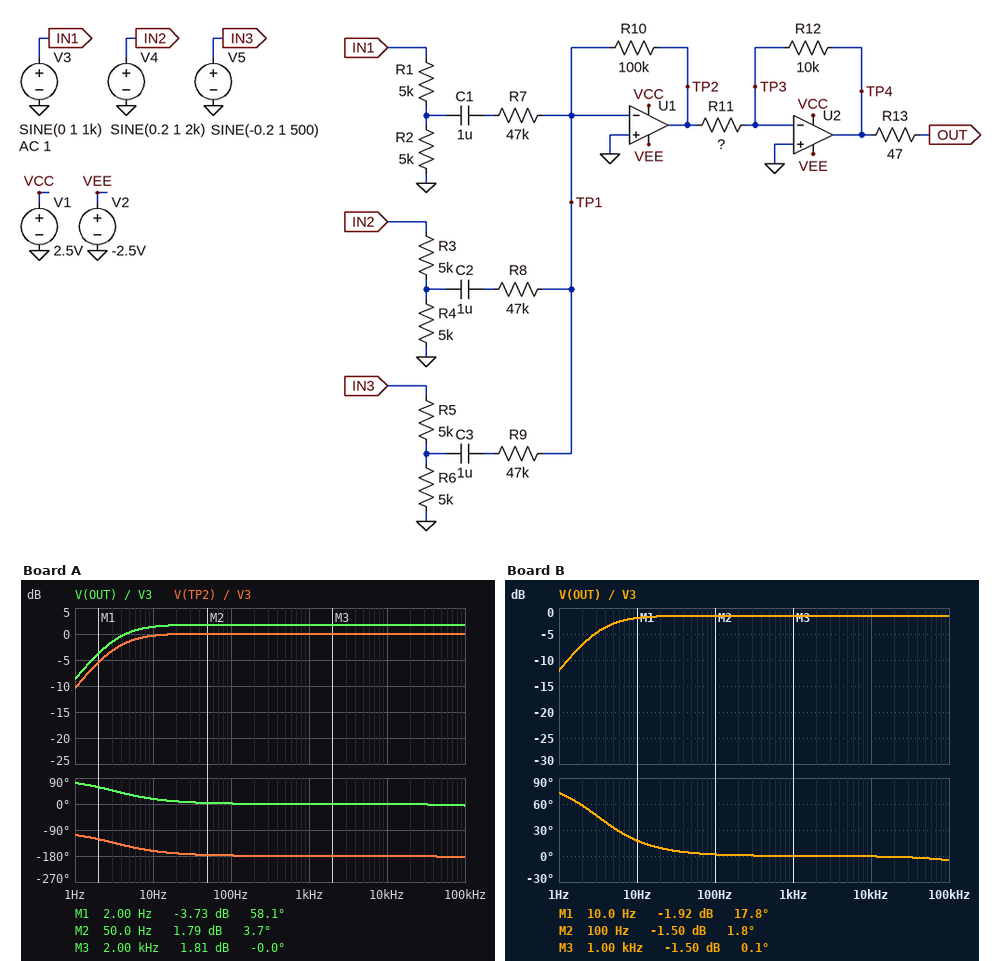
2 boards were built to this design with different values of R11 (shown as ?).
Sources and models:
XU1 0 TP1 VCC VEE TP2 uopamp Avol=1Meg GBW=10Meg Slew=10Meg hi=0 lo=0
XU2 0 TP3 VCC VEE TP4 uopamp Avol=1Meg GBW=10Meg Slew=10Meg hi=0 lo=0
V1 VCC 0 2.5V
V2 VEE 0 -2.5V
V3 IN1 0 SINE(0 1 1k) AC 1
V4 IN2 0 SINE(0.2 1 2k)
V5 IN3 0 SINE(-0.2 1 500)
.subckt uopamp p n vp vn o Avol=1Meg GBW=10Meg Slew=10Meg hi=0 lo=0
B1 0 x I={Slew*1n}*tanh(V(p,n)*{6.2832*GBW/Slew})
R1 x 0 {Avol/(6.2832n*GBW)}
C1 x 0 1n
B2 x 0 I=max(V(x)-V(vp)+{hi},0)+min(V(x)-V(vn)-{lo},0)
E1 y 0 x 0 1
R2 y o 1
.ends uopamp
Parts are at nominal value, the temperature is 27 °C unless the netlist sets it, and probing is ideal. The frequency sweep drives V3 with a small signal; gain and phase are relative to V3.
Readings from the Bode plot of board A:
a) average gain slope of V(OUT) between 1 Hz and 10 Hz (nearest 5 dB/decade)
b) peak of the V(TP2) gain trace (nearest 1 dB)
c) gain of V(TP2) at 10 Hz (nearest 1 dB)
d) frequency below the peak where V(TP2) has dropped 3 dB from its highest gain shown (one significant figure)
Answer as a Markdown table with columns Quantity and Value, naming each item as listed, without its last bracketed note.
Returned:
| Quantity | Value |
|---|---|
| average gain slope of V(OUT) between 1 Hz and 10 Hz | 10 dB/decade |
| peak of the V(TP2) gain trace | 0 dB |
| gain of V(TP2) at 10 Hz | 0 dB |
| frequency below the peak where V(TP2) has dropped 3 dB from its highest gain shown | 3 Hz |
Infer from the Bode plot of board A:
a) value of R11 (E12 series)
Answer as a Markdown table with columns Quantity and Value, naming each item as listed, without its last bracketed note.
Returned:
| Quantity | Value |
|---|---|
| value of R11 | 8.2 kΩ |
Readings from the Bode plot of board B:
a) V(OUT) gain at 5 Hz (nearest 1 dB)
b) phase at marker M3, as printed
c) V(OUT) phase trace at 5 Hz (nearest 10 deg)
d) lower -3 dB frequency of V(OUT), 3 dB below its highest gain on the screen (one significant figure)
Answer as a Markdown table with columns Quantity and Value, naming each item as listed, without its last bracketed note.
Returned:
| Quantity | Value |
|---|---|
| V(OUT) gain at 5 Hz | -3 dB |
| phase at marker M3, as printed | 0.1 deg |
| V(OUT) phase trace at 5 Hz | 30 deg |
| lower -3 dB frequency of V(OUT), 3 dB below its highest gain on the screen | 3 Hz |
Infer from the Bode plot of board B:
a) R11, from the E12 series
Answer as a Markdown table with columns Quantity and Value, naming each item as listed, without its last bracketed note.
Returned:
| Quantity | Value |
|---|---|
| R11, from the E12 series | 12 kΩ |
